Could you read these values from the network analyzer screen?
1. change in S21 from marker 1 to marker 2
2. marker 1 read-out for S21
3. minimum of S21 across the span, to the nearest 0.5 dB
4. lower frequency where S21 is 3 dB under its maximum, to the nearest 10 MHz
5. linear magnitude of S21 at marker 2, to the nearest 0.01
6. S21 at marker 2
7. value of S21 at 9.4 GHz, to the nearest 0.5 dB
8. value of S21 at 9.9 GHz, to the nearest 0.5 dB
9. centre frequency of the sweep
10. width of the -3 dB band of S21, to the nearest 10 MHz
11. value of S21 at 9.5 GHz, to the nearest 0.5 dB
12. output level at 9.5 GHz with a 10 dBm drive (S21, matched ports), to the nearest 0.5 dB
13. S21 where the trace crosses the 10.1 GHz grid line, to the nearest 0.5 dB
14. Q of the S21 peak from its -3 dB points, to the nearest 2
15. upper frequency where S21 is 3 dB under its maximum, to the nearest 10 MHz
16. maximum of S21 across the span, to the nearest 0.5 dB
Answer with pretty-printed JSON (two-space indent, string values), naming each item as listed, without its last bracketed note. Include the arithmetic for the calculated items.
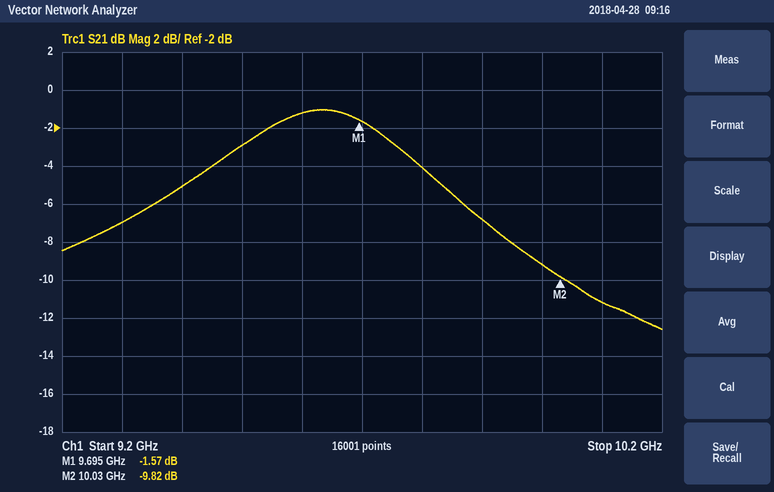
{
  "change in S21 from marker 1 to marker 2": "-9.82 − (-1.57) = -8.25 dB",
  "marker 1 read-out for S21": "-1.57 dB",
  "minimum of S21 across the span, to the nearest 0.5 dB": "-12.5 dB",
  "lower frequency where S21 is 3 dB under its maximum, to the nearest 10 MHz": "9.45 GHz",
  "linear magnitude of S21 at marker 2, to the nearest 0.01": "10^(-9.82/20) ≈ 0.32",
  "S21 at marker 2": "-9.82 dB",
  "value of S21 at 9.4 GHz, to the nearest 0.5 dB": "-5.0 dB",
  "value of S21 at 9.9 GHz, to the nearest 0.5 dB": "-7.0 dB",
  "centre frequency of the sweep": "9.7 GHz",
  "width of the -3 dB band of S21, to the nearest 10 MHz": "9.80 GHz − 9.45 GHz = 350 MHz",
  "value of S21 at 9.5 GHz, to the nearest 0.5 dB": "-3.0 dB",
  "output level at 9.5 GHz with a 10 dBm drive (S21, matched ports), to the nearest 0.5 dB": "10 dBm + (-3.0 dB) = 7.0 dBm",
  "S21 where the trace crosses the 10.1 GHz grid line, to the nearest 0.5 dB": "-11.0 dB",
  "Q of the S21 peak from its -3 dB points, to the nearest 2": "9.625 GHz / 350 MHz ≈ 28",
  "upper frequency where S21 is 3 dB under its maximum, to the nearest 10 MHz": "9.80 GHz",
  "maximum of S21 across the span, to the nearest 0.5 dB": "-1.0 dB"
}
